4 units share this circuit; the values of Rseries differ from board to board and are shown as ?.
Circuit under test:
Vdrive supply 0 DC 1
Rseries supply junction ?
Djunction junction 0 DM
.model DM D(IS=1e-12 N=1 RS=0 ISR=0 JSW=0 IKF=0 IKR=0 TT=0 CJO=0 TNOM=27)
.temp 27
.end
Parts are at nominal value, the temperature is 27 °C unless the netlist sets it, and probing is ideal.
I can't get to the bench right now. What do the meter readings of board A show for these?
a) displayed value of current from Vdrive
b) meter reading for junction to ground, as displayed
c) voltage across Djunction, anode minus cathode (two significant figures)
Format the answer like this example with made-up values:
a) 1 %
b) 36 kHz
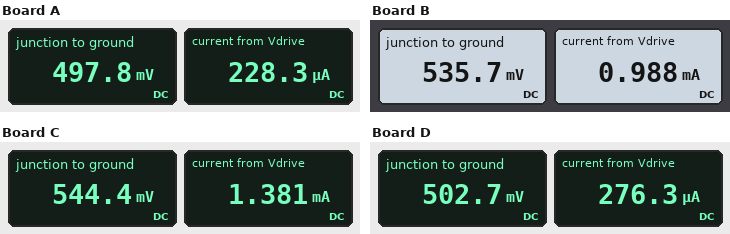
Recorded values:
a) 228.3 µA
b) 497.8 mV
c) 500 mV
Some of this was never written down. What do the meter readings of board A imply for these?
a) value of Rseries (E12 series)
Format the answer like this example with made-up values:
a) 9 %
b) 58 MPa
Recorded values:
a) 2.2 kΩ
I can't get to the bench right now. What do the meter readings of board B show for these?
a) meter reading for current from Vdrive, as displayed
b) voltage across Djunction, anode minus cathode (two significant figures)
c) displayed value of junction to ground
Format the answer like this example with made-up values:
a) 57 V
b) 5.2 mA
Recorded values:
a) 0.988 mA
b) 540 mV
c) 535.7 mV
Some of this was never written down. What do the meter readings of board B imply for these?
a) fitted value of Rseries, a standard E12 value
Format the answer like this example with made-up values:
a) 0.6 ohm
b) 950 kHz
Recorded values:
a) 470 Ω
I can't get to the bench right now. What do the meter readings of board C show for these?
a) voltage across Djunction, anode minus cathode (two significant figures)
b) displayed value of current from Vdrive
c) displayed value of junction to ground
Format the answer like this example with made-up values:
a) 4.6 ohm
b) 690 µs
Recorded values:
a) 540 mV
b) 1.381 mA
c) 544.4 mV
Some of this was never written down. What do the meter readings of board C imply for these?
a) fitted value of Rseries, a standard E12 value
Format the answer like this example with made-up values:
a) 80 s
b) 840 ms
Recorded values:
a) 330 Ω
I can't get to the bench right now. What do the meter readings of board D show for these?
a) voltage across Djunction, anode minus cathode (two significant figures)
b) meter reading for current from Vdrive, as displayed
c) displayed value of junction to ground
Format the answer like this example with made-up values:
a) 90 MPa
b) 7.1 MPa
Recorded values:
a) 500 mV
b) 276.3 µA
c) 502.7 mV
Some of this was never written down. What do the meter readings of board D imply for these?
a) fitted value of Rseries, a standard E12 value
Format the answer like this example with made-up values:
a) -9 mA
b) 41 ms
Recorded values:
a) 1.8 kΩ
